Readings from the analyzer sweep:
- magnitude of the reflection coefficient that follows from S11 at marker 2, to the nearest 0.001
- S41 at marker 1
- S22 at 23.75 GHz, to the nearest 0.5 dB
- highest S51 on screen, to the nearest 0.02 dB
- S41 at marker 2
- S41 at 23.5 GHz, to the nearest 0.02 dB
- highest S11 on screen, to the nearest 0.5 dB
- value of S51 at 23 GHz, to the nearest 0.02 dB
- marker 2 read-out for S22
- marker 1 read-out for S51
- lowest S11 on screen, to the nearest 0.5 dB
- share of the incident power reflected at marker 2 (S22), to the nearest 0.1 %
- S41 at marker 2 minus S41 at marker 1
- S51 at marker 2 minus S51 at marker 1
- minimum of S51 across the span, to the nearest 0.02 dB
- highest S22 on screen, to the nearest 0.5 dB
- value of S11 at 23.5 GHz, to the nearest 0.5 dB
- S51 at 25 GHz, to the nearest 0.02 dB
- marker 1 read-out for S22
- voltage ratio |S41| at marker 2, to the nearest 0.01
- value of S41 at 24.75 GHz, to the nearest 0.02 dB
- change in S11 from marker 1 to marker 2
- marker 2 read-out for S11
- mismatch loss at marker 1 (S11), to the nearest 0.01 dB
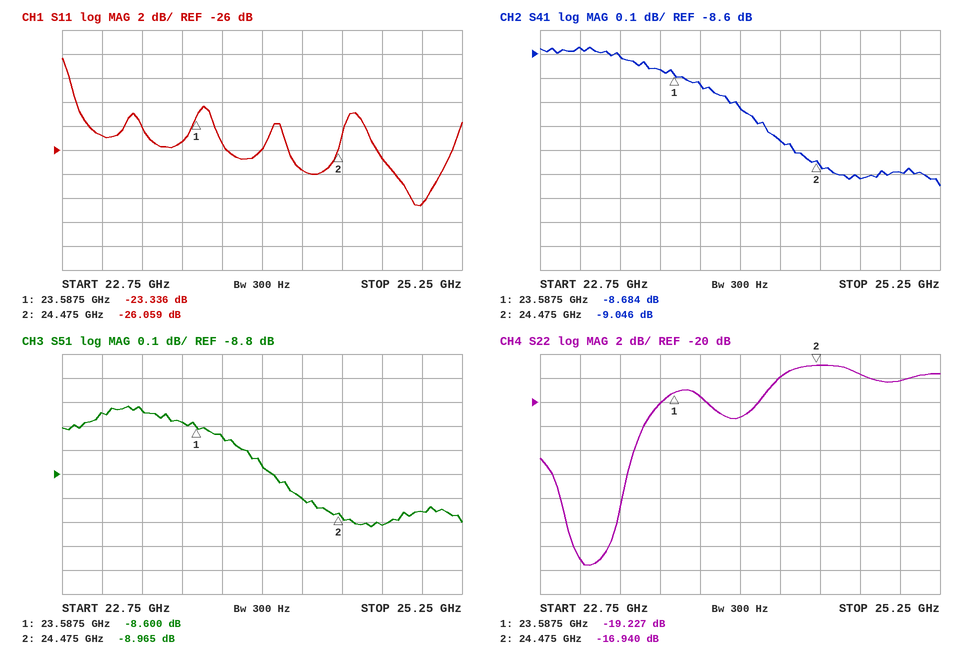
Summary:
0.050
-8.684 dB
-19.5 dB
-8.52 dB
-9.046 dB
-8.66 dB
-18.5 dB
-8.54 dB
-16.940 dB
-8.600 dB
-30.5 dB
2.0 %
-0.362 dB
-0.365 dB
-9.02 dB
-17.0 dB
-25.5 dB
-8.96 dB
-19.227 dB
0.35
-9.12 dB
-2.723 dB
-26.059 dB
0.02 dB
